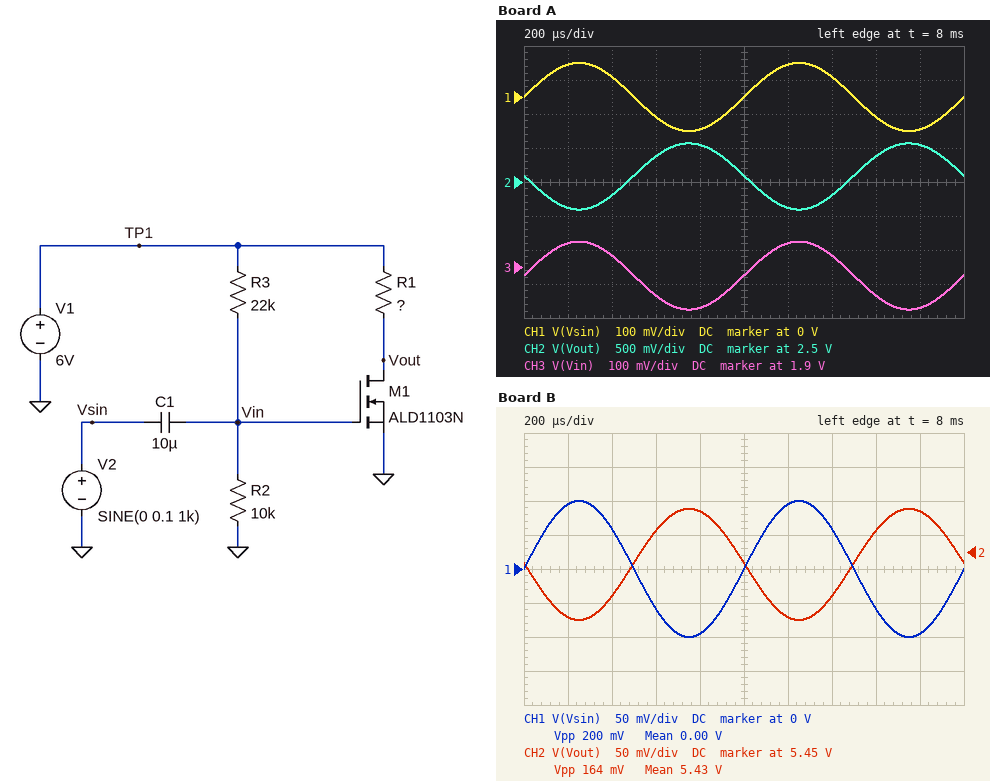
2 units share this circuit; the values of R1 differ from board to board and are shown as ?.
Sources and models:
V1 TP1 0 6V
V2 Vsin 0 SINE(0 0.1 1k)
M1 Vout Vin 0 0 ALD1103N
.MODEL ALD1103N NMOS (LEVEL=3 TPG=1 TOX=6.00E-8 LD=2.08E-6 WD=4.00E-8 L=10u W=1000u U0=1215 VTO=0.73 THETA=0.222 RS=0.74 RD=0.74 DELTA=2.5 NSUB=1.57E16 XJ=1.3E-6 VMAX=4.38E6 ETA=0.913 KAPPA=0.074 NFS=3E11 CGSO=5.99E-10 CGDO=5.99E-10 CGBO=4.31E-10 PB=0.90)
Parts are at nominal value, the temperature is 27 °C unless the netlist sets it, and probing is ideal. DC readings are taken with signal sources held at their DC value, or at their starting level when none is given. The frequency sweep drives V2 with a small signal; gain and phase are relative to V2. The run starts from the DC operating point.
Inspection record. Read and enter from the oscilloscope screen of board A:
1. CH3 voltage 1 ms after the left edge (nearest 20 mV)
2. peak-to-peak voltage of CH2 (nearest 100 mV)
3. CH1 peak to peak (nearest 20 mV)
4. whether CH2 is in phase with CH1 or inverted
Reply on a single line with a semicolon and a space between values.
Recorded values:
1.88 V; 1.0 V; 200 mV; inverted
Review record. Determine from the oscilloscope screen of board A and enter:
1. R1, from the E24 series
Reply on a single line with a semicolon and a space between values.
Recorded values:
680 Ω
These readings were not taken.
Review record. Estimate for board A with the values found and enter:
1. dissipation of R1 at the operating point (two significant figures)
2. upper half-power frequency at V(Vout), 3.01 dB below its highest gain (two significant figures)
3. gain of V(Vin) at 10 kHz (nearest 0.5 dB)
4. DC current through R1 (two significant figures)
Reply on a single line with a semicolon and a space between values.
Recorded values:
17 mW; 420 MHz; 0 dB; 5.0 mA
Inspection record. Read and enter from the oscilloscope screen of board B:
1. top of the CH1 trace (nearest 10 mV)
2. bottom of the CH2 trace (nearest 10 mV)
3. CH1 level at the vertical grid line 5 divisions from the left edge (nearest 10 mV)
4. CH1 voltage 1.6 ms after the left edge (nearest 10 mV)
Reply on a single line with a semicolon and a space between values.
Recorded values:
100 mV; 5.35 V; 0 V; -60 mV
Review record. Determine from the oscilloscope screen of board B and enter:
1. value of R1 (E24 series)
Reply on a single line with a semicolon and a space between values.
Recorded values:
110 Ω
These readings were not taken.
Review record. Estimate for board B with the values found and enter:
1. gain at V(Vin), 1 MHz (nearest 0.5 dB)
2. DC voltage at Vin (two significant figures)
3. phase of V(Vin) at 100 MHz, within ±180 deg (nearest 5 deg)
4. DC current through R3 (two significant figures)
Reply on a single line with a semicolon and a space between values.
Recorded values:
0 dB; 1.9 V; 0 deg; 190 µA
